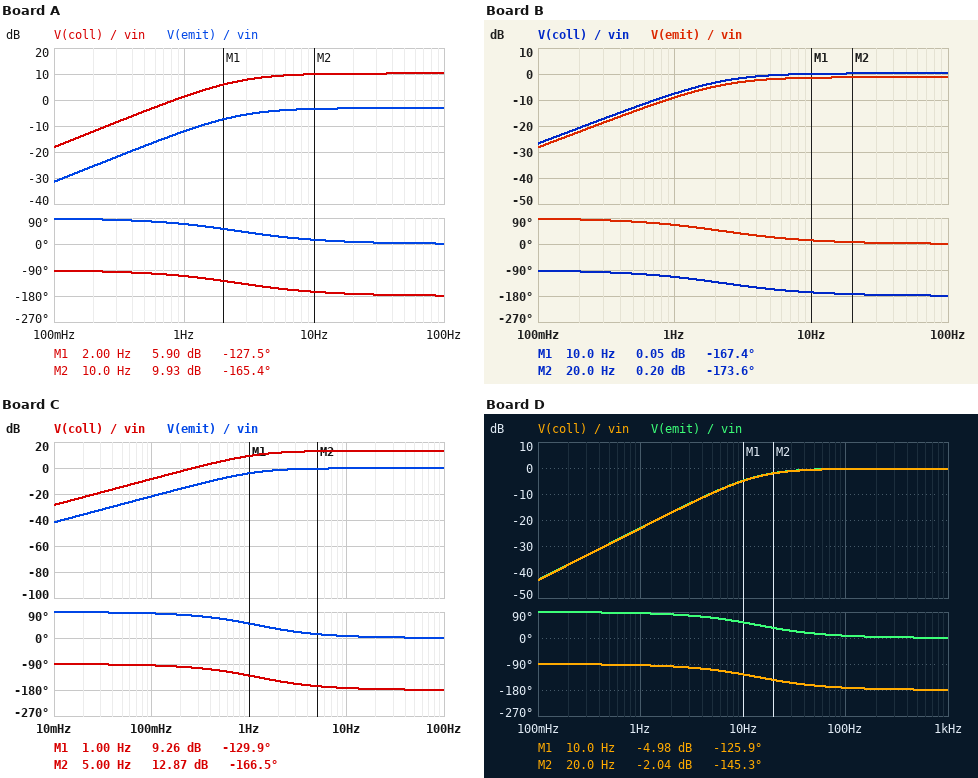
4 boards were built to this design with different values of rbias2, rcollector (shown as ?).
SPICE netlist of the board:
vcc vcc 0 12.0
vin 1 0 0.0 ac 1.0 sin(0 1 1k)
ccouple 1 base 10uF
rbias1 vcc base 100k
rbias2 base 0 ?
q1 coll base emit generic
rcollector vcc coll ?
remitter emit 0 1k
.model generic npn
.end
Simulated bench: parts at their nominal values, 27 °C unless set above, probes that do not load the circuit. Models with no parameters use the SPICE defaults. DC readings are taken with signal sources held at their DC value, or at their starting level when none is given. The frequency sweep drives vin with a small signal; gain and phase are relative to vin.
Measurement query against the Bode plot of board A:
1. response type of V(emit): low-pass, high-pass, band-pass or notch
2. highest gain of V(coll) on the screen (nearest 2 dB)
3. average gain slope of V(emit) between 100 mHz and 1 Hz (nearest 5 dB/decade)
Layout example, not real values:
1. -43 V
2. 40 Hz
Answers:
1. high-pass
2. 10 dB
3. 20 dB/decade
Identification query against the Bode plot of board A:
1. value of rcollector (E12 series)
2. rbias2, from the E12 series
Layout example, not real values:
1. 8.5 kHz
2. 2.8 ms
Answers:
1. 4.7 kΩ
2. 6.8 kΩ
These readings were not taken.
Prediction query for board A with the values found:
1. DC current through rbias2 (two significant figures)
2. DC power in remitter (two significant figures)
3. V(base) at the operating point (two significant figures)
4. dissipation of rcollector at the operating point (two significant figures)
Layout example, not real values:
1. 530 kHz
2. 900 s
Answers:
1. 110 µA
2. 3.5 µW
3. 760 mV
4. 16 µW
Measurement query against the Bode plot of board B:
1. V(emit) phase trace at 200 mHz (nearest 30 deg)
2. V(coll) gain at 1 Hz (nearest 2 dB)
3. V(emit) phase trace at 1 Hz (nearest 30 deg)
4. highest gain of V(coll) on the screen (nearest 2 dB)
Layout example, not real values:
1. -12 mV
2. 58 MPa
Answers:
1. 90 deg
2. -8 dB
3. 60 deg
4. 0 dB
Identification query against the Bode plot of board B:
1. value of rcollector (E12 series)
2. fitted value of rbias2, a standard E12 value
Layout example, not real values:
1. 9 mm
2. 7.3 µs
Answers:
1. 1.2 kΩ
2. 8.2 kΩ
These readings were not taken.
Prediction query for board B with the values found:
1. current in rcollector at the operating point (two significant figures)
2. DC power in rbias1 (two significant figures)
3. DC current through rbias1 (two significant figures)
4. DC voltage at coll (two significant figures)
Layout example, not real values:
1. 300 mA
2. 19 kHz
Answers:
1. 170 µA
2. 1.2 mW
3. 110 µA
4. 12 V
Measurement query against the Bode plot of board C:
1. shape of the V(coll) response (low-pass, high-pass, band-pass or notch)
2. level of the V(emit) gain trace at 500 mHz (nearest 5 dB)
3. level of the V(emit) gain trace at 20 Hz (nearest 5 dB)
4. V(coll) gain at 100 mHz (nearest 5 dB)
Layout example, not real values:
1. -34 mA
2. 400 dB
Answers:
1. high-pass
2. -10 dB
3. 0 dB
4. -10 dB
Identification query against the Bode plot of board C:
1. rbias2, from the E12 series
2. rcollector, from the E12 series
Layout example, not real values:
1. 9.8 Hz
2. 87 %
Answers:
1. 18 kΩ
2. 4.7 kΩ
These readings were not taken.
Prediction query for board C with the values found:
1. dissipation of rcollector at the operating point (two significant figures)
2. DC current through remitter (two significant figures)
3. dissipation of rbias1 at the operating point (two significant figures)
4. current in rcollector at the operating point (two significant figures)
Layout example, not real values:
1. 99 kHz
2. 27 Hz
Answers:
1. 3.9 mW
2. 920 µA
3. 1.1 mW
4. 910 µA
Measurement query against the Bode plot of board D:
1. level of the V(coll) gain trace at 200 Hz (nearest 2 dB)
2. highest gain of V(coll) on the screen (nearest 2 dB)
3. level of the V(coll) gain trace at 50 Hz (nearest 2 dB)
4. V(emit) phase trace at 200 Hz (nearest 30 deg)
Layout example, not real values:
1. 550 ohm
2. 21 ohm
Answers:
1. 0 dB
2. 0 dB
3. 0 dB
4. 0 deg
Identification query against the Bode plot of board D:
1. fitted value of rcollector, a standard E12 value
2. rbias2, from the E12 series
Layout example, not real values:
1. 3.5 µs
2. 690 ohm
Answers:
1. 6.8 kΩ
2. 33 kΩ
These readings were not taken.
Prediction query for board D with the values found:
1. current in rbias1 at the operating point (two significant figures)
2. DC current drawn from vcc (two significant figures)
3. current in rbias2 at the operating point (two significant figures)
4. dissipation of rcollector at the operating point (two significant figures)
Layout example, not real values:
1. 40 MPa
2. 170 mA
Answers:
1. 97 µA
2. 1.6 mA
3. 71 µA
4. 16 mW
